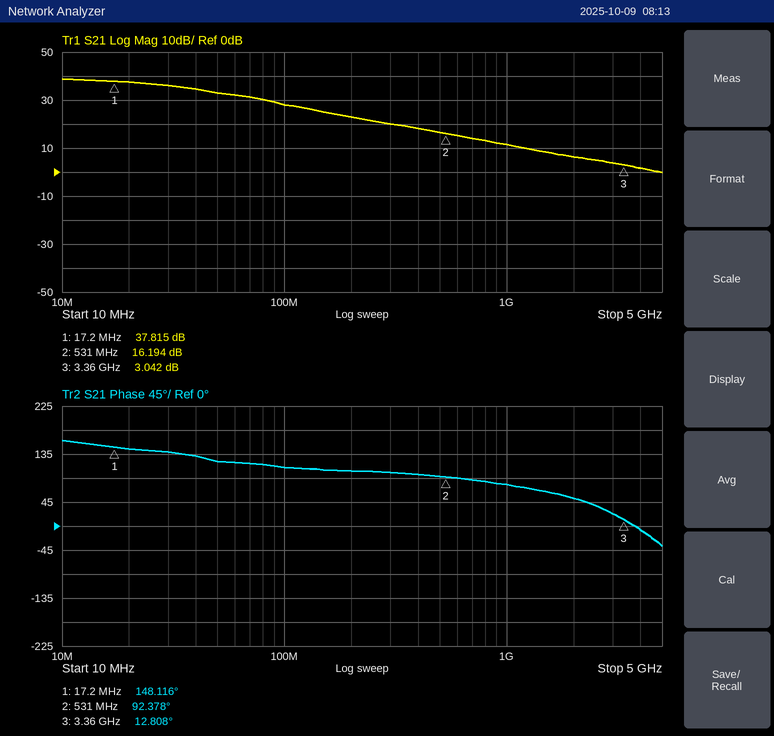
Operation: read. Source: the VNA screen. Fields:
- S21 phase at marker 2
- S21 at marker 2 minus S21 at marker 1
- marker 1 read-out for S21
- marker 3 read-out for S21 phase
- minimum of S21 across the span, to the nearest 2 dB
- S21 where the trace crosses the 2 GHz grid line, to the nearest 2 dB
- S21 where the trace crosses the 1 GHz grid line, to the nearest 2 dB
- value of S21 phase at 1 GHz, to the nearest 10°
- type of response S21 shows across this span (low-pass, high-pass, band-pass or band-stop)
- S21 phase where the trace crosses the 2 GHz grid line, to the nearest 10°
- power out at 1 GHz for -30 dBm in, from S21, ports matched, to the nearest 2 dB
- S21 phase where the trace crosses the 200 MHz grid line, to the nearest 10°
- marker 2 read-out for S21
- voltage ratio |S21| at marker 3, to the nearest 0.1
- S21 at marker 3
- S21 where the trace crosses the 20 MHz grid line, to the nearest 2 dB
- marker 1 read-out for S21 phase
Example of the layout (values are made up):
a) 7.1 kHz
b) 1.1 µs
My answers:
a) 92.378°
b) -21.621 dB
c) 37.815 dB
d) 12.808°
e) 0 dB
f) 6 dB
g) 12 dB
h) 80°
i) low-pass
j) 50°
k) -18 dBm
l) 100°
m) 16.194 dB
n) 1.4
o) 3.042 dB
p) 38 dB
q) 148.116°
